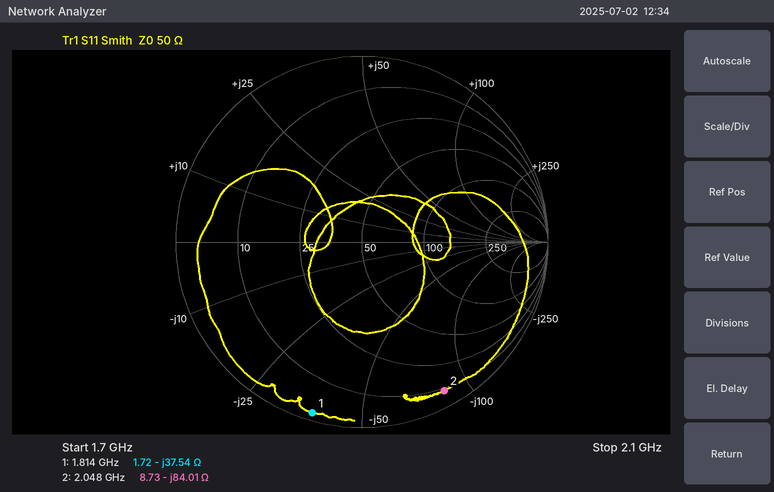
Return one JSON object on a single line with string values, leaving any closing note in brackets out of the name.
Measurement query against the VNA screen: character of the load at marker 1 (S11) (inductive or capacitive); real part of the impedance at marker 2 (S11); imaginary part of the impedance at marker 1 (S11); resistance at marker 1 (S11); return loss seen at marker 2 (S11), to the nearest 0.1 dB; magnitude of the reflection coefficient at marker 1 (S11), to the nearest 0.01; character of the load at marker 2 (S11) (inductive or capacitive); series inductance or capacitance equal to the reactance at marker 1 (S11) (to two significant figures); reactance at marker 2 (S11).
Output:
{"character of the load at marker 1 (S11)": "capacitive", "real part of the impedance at marker 2": "8.73 Ω", "imaginary part of the impedance at marker 1": "-37.54 Ω", "resistance at marker 1": "1.72 Ω", "return loss seen at marker 2 (S11), to the nearest 0.1 dB": "0.8 dB", "magnitude of the reflection coefficient at marker 1 (S11), to the nearest 0.01": "0.96", "character of the load at marker 2 (S11)": "capacitive", "series inductance or capacitance equal to the reactance at marker 1 (S11)": "2.3 pF", "reactance at marker 2": "-84.01 Ω"}
